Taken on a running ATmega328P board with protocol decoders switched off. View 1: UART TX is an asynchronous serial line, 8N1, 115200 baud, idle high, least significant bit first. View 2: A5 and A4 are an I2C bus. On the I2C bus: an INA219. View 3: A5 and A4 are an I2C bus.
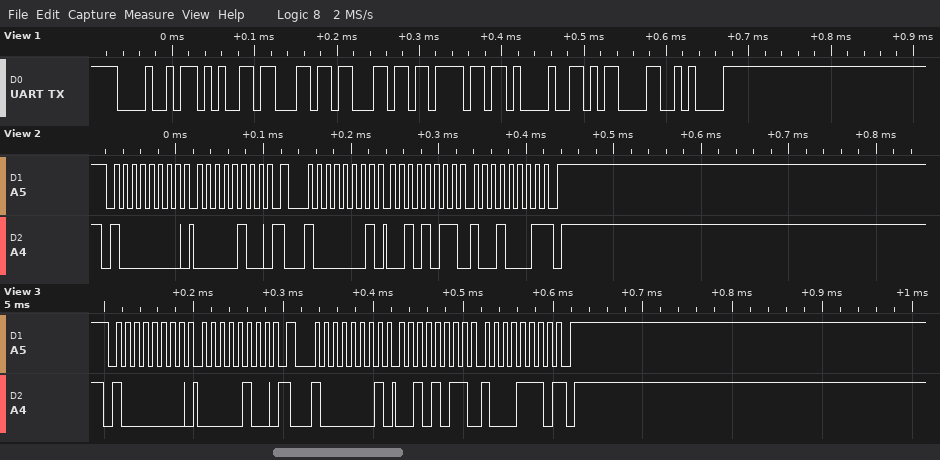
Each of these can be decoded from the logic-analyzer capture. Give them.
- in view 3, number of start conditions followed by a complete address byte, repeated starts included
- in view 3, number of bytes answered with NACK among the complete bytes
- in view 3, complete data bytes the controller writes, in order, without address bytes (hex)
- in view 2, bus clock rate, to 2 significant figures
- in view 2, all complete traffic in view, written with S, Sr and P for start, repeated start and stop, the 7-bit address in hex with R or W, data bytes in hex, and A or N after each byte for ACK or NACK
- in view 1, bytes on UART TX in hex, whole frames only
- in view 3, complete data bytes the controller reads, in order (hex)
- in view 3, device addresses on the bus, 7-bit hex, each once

2
1
04
100 kHz
S 40W A 04 A Sr 40R A 2B A 91 N P
48 65 6C 6C 6F 21 0D 0A
2B 8E
0x40
